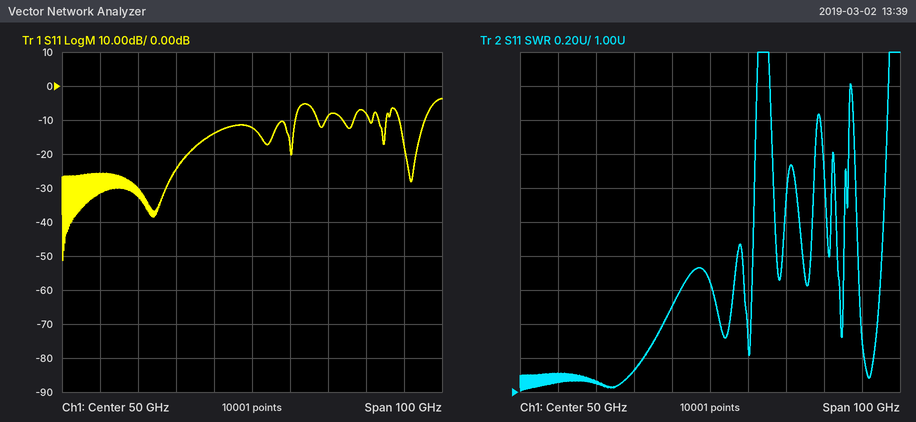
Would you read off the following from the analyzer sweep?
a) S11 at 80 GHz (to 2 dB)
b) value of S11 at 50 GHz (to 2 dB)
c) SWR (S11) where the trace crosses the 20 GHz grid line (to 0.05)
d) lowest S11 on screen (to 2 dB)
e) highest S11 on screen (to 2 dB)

-8 dB
-12 dB
1.05
-52 dB
-4 dB
